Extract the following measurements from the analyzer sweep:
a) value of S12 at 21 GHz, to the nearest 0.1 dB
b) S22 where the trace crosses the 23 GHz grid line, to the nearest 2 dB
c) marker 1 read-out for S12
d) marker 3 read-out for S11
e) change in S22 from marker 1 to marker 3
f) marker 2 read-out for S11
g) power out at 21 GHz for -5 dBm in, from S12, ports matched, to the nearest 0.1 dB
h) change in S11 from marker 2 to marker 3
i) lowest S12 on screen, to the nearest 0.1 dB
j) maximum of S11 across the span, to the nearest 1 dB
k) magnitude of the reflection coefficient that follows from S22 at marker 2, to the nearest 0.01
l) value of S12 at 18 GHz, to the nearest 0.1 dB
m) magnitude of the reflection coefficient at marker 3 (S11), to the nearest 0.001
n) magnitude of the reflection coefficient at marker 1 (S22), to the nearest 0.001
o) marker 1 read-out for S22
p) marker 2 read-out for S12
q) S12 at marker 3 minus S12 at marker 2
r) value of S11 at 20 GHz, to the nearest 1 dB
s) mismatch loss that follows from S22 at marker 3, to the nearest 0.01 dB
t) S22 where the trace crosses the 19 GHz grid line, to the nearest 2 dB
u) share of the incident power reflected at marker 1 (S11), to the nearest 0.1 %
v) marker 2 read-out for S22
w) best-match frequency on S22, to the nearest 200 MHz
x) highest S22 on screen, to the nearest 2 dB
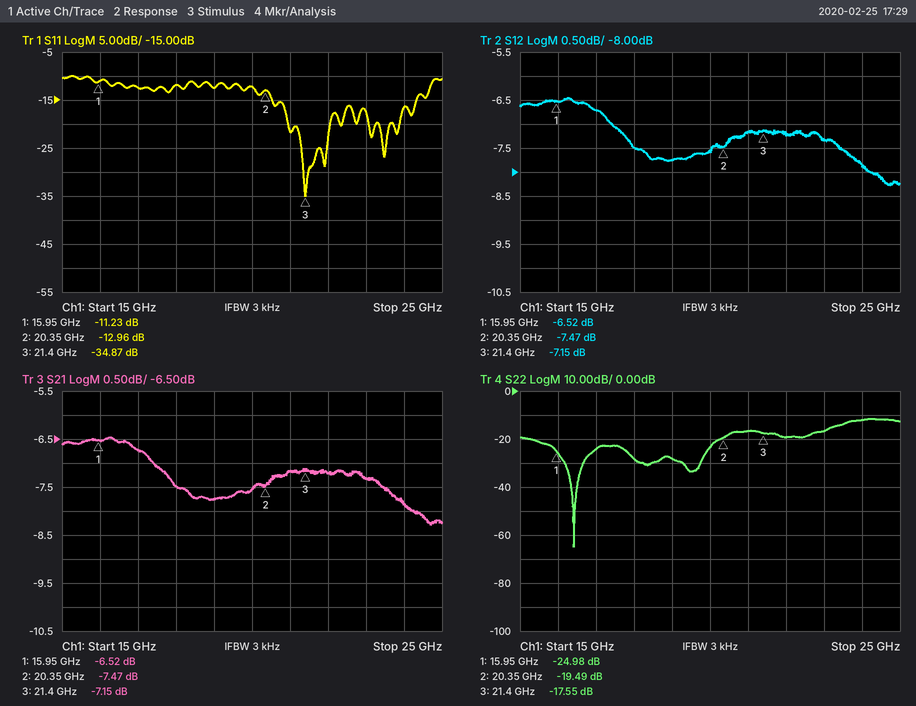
-7.2 dB
-16 dB
-6.52 dB
-34.87 dB
7.43 dB
-12.96 dB
-12.2 dBm
-21.91 dB
-8.3 dB
-10 dB
0.11
-7.5 dB
0.018
0.056
-24.98 dB
-7.47 dB
0.32 dB
-12 dB
0.08 dB
-28 dB
7.5 %
-19.49 dB
16.4 GHz
-12 dB
